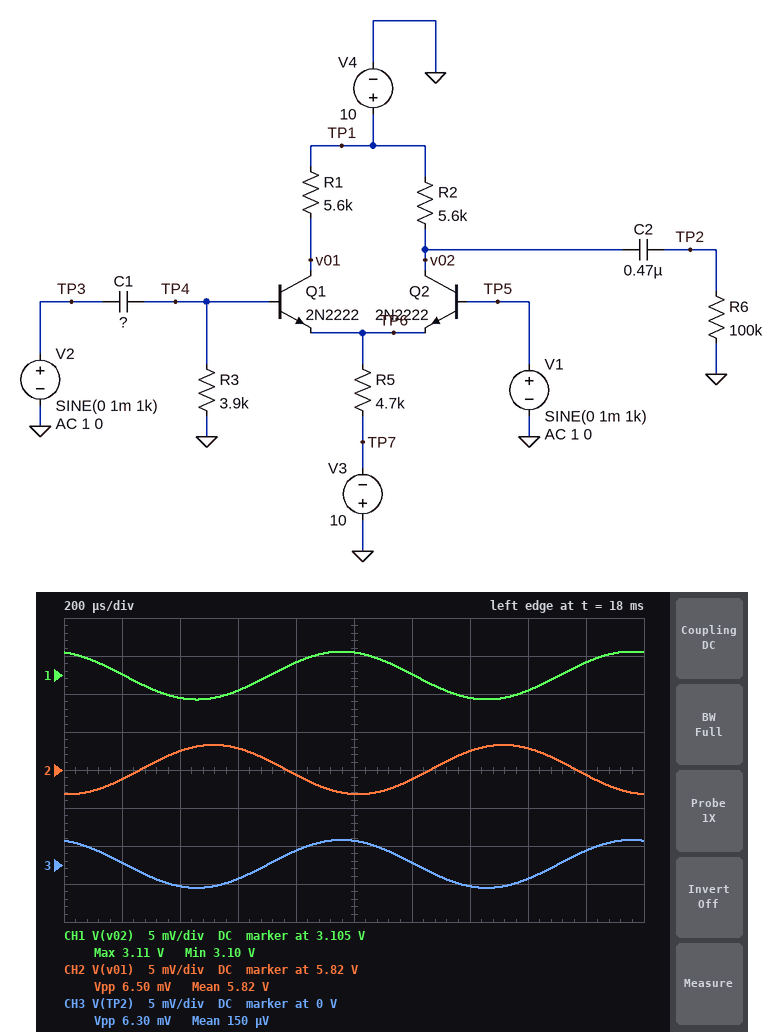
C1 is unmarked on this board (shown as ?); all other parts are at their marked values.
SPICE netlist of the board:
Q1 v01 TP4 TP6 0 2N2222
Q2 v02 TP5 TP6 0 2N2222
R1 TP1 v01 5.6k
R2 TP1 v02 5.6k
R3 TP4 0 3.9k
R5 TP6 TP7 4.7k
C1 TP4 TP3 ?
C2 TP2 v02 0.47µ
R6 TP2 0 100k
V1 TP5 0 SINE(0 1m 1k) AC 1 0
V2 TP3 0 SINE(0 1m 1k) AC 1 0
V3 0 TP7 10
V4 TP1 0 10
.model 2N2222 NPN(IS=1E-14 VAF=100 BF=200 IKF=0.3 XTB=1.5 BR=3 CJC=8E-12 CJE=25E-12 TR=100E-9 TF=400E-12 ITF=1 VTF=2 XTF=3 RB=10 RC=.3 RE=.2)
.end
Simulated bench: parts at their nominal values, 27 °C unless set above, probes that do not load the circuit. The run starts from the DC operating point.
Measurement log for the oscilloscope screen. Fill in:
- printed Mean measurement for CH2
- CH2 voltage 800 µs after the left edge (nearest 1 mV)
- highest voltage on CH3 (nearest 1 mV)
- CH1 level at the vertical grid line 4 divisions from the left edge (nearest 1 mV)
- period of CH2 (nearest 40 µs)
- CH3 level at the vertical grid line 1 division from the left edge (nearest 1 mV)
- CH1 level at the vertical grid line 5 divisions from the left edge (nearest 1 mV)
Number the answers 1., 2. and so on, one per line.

1. 5.82 V
2. 5.819 V
3. 3 mV
4. 3.107 V
5. 1.00 ms
6. 0 V
7. 3.108 V
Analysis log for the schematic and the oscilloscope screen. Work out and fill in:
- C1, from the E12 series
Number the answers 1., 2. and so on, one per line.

1. 1.2 µF
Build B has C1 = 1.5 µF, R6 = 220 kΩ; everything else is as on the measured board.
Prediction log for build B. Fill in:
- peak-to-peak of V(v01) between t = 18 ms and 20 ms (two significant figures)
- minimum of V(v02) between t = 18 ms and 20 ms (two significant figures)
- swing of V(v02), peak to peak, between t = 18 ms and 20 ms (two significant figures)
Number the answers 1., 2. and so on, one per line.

1. 5.2 mV
2. 3.1 V
3. 5.3 mV
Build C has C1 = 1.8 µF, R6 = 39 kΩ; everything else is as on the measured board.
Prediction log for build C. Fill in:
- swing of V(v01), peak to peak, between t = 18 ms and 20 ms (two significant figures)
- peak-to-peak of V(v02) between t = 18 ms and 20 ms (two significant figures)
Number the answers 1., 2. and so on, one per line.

1. 4.4 mV
2. 4.0 mV
